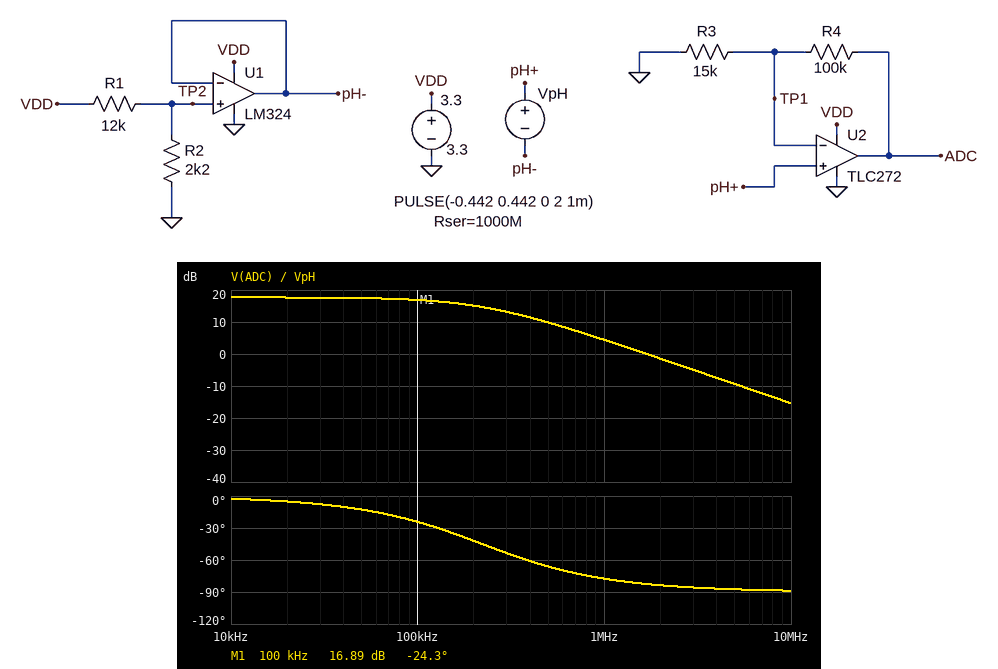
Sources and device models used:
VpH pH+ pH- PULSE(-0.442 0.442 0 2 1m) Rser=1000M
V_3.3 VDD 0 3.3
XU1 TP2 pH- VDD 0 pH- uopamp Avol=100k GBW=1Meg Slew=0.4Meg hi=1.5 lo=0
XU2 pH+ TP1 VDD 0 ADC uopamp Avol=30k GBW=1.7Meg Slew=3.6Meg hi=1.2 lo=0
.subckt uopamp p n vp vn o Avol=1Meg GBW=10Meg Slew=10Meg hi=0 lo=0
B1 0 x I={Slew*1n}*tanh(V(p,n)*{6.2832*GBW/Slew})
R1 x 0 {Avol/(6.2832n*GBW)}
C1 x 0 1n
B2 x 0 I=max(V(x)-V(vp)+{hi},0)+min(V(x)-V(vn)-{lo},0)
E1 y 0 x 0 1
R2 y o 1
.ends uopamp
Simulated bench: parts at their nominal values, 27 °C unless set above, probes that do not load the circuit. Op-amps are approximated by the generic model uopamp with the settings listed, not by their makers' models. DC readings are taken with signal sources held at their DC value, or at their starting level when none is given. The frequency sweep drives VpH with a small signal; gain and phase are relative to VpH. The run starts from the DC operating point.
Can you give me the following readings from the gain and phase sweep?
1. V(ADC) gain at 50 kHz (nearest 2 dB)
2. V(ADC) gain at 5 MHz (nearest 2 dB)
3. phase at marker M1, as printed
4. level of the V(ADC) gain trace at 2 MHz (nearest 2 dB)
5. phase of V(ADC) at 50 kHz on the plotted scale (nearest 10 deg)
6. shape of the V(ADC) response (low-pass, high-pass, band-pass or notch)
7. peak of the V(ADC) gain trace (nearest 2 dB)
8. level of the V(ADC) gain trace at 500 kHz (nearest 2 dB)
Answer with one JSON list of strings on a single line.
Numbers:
["18 dB", "-10 dB", "-24.3 deg", "-2 dB", "-10 deg", "low-pass", "18 dB", "10 dB"]
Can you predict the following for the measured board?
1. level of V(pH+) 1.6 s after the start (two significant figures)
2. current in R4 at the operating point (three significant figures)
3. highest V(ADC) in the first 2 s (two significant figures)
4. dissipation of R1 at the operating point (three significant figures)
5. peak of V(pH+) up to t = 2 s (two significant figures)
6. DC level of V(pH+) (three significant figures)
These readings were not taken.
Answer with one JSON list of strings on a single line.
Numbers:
["780 mV", "4.62 µA", "2.1 V", "648 µW", "950 mV", "69.3 mV"]
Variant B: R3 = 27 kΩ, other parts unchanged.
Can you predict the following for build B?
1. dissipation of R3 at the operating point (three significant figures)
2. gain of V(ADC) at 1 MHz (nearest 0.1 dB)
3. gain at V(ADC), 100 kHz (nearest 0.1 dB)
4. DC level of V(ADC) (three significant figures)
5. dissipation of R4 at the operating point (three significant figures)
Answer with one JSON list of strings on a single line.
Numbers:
["178 nW", "4.1 dB", "13.1 dB", "326 mV", "658 nW"]
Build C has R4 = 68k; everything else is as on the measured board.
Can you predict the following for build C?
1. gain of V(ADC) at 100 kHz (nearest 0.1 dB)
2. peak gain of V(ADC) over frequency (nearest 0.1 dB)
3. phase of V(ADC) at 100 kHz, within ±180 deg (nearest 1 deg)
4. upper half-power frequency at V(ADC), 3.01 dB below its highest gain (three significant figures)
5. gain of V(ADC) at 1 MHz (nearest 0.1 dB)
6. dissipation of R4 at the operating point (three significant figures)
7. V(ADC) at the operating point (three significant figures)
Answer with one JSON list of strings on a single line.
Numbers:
["14.4 dB", "14.9 dB", "-18 deg", "307 kHz", "4.2 dB", "1.45 µW", "383 mV"]
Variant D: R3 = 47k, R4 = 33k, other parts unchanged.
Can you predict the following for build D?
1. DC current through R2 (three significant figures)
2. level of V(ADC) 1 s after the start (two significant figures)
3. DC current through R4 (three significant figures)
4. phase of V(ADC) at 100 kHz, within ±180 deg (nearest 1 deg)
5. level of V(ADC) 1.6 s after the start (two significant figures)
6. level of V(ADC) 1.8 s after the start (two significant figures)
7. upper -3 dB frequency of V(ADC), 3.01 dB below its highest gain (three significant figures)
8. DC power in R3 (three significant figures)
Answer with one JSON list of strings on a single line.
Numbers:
["232 µA", "870 mV", "1.47 µA", "-6 deg", "1.3 V", "1.5 V", "999 kHz", "102 nW"]
